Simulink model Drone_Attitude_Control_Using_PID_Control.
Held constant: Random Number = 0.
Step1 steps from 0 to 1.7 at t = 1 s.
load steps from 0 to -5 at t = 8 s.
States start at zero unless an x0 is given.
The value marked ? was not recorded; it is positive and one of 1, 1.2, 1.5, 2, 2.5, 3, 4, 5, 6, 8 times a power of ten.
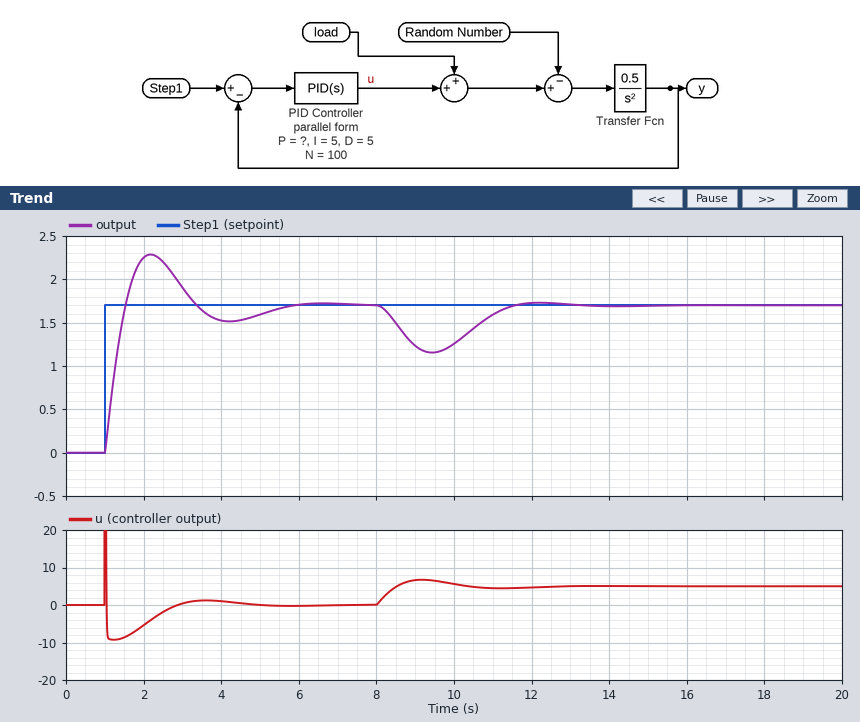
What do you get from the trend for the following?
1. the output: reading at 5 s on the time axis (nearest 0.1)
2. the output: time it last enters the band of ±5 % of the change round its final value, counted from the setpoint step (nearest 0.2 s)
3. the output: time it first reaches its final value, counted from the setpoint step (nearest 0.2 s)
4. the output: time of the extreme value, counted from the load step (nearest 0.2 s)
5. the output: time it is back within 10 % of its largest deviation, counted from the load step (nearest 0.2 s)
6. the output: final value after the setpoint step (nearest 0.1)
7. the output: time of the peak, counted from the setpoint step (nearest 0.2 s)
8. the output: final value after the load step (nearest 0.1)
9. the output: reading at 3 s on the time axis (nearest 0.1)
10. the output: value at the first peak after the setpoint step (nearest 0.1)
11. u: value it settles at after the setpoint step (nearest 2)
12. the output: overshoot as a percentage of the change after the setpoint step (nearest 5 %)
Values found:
1.6
4.2 s
0.6 s
1.4 s
3.2 s
1.7
1.2 s
1.7
1.9
2.3
0
35 %
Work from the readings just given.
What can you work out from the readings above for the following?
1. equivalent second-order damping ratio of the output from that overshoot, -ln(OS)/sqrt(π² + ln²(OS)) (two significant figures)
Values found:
0.32
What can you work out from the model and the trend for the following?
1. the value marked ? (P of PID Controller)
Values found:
8
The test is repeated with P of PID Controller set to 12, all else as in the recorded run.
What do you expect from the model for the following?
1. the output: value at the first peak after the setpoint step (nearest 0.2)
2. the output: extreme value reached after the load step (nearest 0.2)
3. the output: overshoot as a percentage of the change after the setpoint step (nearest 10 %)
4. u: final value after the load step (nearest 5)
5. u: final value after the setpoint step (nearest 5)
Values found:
2.4
1.2
40 %
5
0
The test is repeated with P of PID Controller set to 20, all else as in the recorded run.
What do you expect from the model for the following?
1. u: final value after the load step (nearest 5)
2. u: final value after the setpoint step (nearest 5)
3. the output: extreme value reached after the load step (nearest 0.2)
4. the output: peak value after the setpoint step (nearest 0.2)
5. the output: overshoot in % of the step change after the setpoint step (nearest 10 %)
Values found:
5
0
1.4
2.4
40 %
